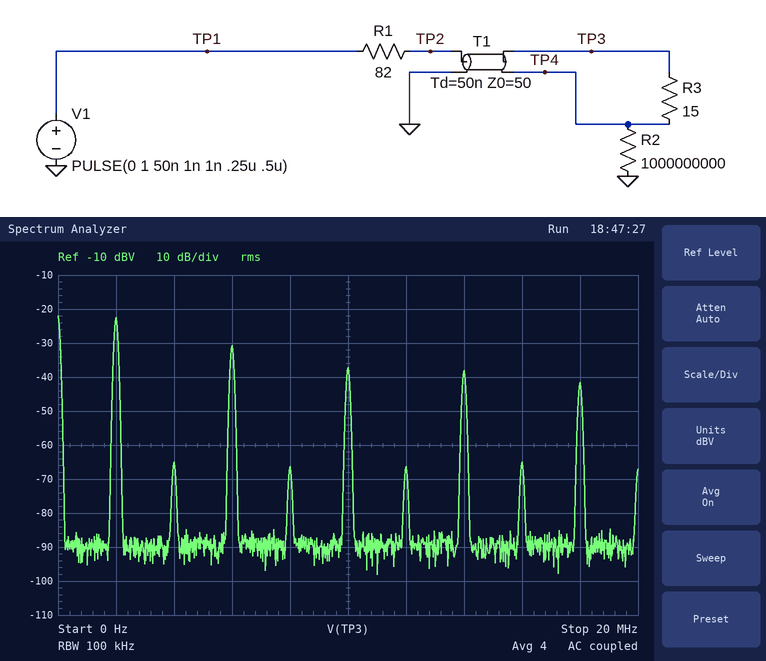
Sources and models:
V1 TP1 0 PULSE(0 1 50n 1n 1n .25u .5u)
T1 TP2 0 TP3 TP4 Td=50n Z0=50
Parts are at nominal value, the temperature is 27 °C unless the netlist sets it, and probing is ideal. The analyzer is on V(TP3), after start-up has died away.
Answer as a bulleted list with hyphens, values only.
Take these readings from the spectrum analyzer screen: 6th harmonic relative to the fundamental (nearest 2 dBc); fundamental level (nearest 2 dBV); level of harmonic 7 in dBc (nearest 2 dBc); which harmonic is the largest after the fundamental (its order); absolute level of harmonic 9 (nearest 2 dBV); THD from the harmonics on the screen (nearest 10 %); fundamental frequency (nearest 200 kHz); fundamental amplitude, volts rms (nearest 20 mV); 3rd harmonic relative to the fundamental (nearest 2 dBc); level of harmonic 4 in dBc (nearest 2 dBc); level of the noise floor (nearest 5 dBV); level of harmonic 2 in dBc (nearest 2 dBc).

- -44 dBc
- -22 dBV
- -16 dBc
- 3
- -42 dBV
- 50 %
- 2.0 MHz
- 80 mV
- -8 dBc
- -44 dBc
- -90 dBV
- -42 dBc
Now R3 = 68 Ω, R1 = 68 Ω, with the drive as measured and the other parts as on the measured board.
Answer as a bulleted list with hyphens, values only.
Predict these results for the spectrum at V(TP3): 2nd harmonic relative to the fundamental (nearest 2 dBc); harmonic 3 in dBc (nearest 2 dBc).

- -44 dBc
- -10 dBc
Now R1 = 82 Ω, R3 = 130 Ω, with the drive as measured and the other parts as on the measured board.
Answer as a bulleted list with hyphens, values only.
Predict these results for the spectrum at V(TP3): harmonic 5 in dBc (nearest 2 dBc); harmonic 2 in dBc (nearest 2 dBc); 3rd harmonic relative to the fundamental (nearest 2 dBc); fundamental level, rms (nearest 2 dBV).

- -14 dBc
- -46 dBc
- -10 dBc
- -12 dBV
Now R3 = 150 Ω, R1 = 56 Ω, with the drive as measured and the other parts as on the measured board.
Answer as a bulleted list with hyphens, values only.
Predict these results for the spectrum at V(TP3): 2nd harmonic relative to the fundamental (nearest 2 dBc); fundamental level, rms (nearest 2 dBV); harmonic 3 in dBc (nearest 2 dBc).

- -44 dBc
- -10 dBV
- -10 dBc
